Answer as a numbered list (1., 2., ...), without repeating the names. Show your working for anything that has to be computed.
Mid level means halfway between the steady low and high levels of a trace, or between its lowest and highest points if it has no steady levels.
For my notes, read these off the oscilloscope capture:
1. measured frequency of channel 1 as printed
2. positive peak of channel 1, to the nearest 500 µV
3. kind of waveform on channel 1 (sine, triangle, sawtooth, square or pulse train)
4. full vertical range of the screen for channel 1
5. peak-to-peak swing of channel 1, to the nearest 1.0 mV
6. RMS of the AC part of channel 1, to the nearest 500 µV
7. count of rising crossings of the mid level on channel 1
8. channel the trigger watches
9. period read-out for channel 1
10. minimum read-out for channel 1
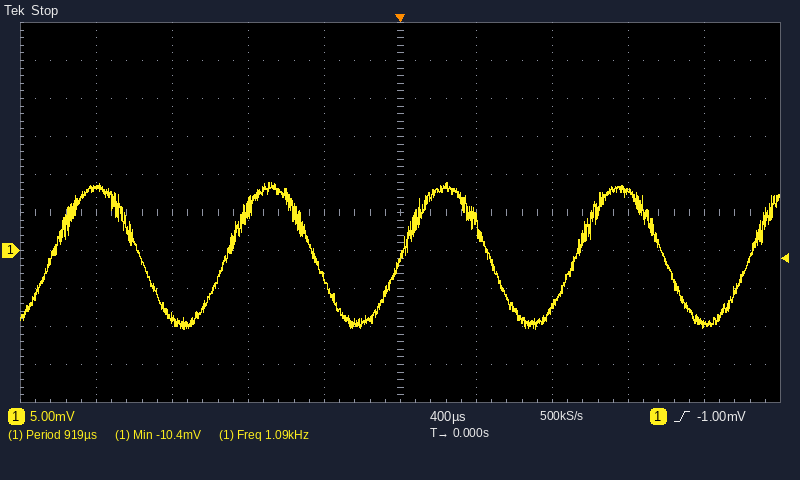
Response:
1. 1.09 kHz
2. 9.0 mV
3. sine
4. 50 mV
5. 19.0 mV
6. 19.0 mV / (2√2) ≈ 6.72 mV, so 6.5 mV to the nearest 500 µV
7. 5
8. channel 1
9. 919 µs
10. -10.4 mV
